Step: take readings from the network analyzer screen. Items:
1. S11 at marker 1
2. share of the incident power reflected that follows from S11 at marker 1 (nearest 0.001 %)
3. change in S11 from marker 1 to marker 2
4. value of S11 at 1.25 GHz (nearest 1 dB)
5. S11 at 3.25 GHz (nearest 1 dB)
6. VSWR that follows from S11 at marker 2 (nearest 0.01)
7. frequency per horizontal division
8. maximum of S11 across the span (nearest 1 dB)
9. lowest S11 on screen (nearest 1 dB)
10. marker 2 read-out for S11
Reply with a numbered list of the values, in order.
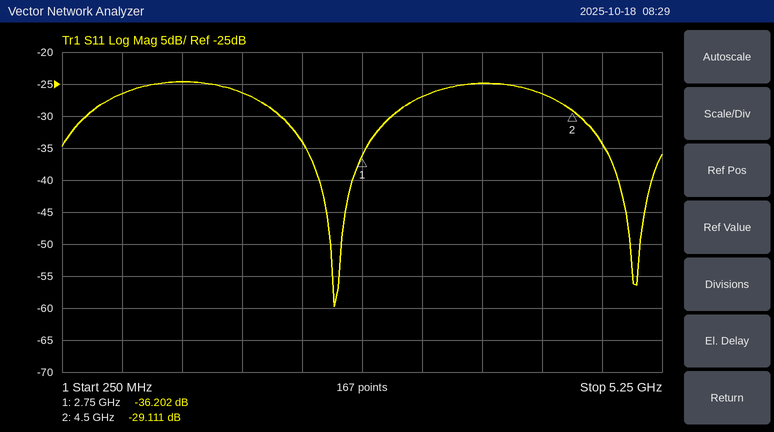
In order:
1. -36.202 dB
2. 0.024 %
3. 7.091 dB
4. -25 dB
5. -27 dB
6. 1.07
7. 500 MHz
8. -25 dB
9. -60 dB
10. -29.111 dB
